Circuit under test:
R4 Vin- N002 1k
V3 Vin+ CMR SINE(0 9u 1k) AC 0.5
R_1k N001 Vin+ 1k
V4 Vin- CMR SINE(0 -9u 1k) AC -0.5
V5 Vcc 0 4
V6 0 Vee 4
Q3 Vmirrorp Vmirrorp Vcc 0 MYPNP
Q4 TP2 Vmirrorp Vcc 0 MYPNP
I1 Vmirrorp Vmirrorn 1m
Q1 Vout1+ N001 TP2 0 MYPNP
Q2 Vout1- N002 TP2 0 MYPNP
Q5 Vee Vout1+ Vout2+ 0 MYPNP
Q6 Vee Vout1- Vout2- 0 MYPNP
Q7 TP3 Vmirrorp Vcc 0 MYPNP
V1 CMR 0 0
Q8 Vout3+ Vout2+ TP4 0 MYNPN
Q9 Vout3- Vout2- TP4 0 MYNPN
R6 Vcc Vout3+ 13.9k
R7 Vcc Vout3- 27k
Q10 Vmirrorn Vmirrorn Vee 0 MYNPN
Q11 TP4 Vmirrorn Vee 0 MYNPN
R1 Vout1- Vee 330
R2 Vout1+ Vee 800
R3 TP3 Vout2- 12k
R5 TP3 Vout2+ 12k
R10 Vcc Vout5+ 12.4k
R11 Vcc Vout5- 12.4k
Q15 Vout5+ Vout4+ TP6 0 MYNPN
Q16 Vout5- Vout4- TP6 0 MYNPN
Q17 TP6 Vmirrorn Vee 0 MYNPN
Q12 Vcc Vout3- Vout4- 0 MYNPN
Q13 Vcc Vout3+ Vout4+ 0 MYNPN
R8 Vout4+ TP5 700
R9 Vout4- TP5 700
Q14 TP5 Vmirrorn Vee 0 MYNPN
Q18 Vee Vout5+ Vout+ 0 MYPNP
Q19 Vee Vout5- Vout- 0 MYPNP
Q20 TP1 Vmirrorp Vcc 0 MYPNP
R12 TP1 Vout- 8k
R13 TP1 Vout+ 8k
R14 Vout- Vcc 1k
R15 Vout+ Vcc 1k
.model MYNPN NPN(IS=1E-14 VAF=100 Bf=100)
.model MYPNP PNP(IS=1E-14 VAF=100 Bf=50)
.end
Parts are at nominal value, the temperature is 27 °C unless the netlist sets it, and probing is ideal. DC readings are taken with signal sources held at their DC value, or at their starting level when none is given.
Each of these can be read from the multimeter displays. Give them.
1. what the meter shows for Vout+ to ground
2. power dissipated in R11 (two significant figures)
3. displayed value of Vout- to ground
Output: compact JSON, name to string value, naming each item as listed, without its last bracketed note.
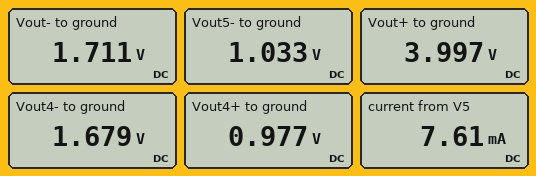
{"what the meter shows for Vout+ to ground": "3.997 V", "power dissipated in R11": "710 µW", "displayed value of Vout- to ground": "1.711 V"}
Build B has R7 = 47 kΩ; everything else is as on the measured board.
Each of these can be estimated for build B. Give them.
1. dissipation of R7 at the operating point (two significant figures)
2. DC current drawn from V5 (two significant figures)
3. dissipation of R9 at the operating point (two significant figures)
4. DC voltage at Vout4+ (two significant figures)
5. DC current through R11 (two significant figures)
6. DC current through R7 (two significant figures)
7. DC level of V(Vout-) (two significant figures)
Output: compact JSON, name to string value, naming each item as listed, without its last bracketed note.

{"dissipation of R7 at the operating point": "120 µW", "DC current drawn from V5": "8.4 mA", "dissipation of R9 at the operating point": "690 µW", "DC voltage at Vout4+": "270 mV", "DC current through R11": "300 µA", "DC current through R7": "50 µA", "DC level of V(Vout-)": "1.0 V"}
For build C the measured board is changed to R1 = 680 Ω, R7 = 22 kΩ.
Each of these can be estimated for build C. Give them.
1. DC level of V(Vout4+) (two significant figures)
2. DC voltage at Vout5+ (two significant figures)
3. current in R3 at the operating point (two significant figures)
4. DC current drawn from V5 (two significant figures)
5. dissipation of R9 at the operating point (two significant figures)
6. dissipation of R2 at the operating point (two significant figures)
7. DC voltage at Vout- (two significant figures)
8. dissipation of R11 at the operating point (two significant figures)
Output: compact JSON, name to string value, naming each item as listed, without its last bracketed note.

{"DC level of V(Vout4+)": "-2.6 V", "DC voltage at Vout5+": "4.0 V", "current in R3 at the operating point": "440 µA", "DC current drawn from V5": "12 mA", "dissipation of R9 at the operating point": "660 µW", "dissipation of R2 at the operating point": "150 µW", "DC voltage at Vout-": "-1.8 V", "dissipation of R11 at the operating point": "3.4 mW"}
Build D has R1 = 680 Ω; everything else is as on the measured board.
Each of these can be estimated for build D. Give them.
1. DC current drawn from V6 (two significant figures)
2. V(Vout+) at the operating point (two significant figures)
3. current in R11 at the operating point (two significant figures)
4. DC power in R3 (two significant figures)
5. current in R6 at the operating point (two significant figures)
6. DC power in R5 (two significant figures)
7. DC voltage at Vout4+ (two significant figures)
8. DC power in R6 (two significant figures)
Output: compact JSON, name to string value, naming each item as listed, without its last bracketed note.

{"DC current drawn from V6": "13 mA", "V(Vout+) at the operating point": "4.0 V", "current in R11 at the operating point": "600 µA", "DC power in R3": "2.5 mW", "current in R6 at the operating point": "550 µA", "DC power in R5": "2.4 mW", "DC voltage at Vout4+": "-3.5 V", "DC power in R6": "4.2 mW"}
